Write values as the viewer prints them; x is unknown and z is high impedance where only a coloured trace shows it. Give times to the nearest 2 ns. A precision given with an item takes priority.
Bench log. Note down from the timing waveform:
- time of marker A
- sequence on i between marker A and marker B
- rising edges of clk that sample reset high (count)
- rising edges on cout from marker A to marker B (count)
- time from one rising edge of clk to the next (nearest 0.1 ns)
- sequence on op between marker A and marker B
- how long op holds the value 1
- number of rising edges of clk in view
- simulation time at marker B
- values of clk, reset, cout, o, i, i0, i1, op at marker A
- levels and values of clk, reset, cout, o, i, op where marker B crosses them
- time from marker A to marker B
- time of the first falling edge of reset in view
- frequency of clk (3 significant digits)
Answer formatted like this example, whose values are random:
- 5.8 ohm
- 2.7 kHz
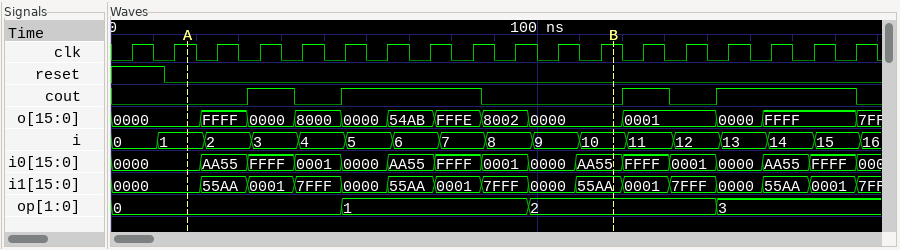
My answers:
- 18 ns
- 1, 2, 3, 4, 5, 6, 7, 8, 9, 10
- 1
- 2
- 10 ns
- 0, 1, 2
- 44 ns
- 18
- 118 ns
- clk=1, reset=0, cout=0, o=0000, i=1, i0=0000, i1=0000, op=0
- clk=1, reset=0, cout=0, o=0000, i=10, op=2
- 100 ns
- 12 ns
- 100 MHz
